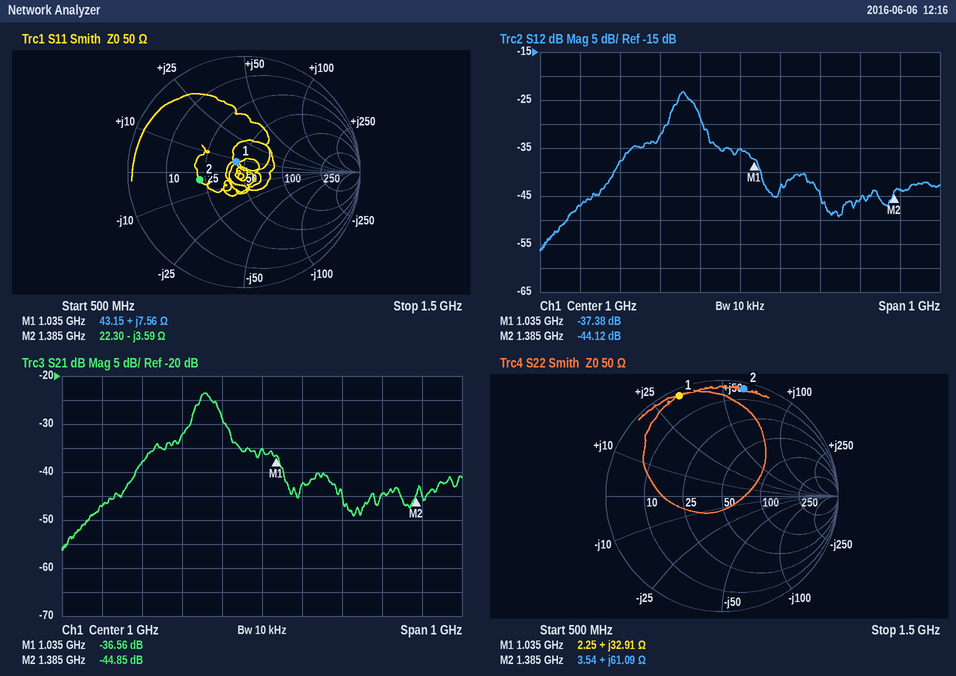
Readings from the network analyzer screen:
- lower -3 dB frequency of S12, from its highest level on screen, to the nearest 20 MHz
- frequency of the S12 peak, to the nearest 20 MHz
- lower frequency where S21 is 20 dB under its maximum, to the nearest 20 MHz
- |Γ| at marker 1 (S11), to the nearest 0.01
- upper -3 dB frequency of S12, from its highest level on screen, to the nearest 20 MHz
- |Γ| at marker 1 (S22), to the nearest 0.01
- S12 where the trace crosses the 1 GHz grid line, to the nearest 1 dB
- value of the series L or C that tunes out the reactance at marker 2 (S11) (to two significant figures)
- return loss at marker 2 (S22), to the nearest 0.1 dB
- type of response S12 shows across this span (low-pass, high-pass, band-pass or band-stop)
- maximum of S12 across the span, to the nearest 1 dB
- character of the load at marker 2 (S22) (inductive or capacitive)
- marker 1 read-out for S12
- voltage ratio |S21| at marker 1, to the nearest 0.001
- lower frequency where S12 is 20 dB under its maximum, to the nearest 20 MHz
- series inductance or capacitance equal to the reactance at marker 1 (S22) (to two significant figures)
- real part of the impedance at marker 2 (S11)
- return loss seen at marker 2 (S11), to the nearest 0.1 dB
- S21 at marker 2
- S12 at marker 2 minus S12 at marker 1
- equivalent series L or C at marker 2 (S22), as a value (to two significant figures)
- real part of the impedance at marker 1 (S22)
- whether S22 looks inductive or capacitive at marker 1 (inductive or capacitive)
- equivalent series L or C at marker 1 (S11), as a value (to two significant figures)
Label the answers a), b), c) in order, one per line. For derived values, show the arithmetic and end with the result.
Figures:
a) 840 MHz
b) 860 MHz
c) 660 MHz
d) 0.11
e) 880 MHz
f) 0.94
g) -35 dB
h) L = 3.59 Ω/(2π × 1.385 GHz) ≈ 413 pH, so 410 pH to two significant figures
i) 0.5 dB
j) band-pass
k) -23 dB
l) inductive
m) -37.38 dB
n) 10^(-36.56/20) ≈ 0.015
o) 660 MHz
p) L = 32.91 Ω/(2π × 1.035 GHz) ≈ 5.1 nH
q) 22.30 Ω
r) 8.3 dB
s) -44.85 dB
t) -44.12 − (-37.38) = -6.74 dB
u) L = 61.09 Ω/(2π × 1.385 GHz) ≈ 7.0 nH
v) 2.25 Ω
w) inductive
x) L = 7.56 Ω/(2π × 1.035 GHz) ≈ 1.2 nH
